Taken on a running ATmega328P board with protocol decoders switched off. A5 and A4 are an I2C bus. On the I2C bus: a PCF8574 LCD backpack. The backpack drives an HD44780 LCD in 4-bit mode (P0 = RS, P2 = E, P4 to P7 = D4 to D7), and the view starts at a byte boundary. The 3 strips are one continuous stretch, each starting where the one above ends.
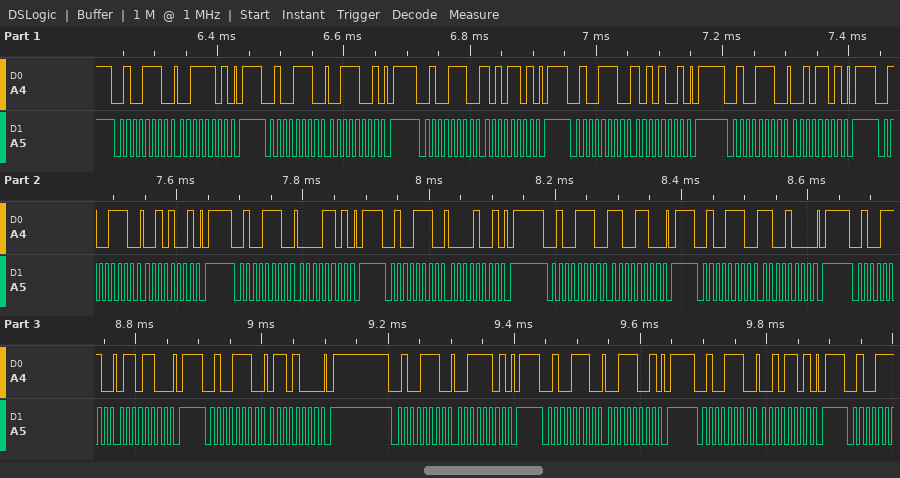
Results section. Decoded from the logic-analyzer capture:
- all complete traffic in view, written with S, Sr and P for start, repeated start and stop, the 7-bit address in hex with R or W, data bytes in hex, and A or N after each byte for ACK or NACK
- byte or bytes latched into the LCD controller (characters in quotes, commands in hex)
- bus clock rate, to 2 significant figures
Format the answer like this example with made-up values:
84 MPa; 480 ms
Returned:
S 27W A 3D A P S 27W A 39 A P S 27W A AD A P S 27W A A9 A P S 27W A 2D A P S 27W A 29 A P S 27W A 0D A P S 27W A 09 A P S 27W A CC A P S 27W A C8 A P S 27W A 6C A P S 27W A 68 A P S 27W A 3D A P S 27W A 39 A P S 27W A 2D A P; ':' ' ' 0xC6; 100 kHz
